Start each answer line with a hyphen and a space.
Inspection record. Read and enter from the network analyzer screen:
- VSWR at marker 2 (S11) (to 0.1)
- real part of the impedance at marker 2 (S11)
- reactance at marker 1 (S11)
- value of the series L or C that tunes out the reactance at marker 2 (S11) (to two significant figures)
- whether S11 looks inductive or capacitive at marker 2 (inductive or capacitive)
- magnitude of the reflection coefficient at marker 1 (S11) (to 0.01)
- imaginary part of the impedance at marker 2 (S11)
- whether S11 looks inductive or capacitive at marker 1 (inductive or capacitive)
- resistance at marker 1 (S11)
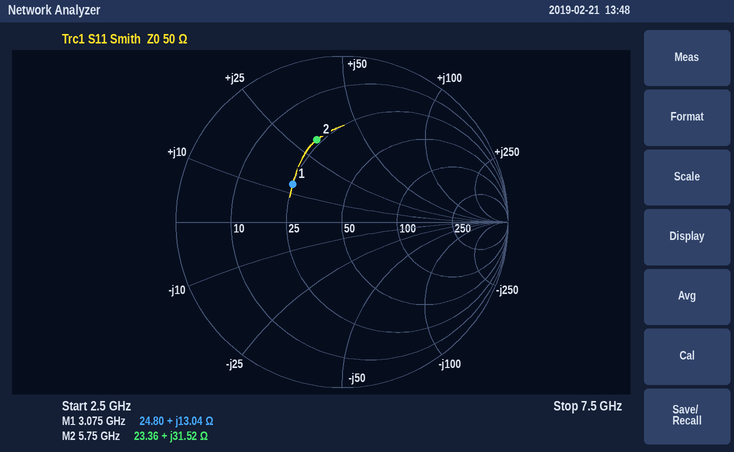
- 3.1
- 23.36 Ω
- +13.04 Ω
- 880 fF
- inductive
- 0.37
- +31.52 Ω
- inductive
- 24.80 Ω
